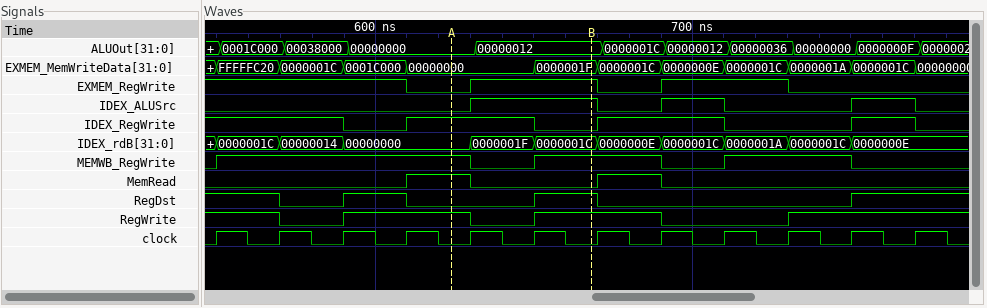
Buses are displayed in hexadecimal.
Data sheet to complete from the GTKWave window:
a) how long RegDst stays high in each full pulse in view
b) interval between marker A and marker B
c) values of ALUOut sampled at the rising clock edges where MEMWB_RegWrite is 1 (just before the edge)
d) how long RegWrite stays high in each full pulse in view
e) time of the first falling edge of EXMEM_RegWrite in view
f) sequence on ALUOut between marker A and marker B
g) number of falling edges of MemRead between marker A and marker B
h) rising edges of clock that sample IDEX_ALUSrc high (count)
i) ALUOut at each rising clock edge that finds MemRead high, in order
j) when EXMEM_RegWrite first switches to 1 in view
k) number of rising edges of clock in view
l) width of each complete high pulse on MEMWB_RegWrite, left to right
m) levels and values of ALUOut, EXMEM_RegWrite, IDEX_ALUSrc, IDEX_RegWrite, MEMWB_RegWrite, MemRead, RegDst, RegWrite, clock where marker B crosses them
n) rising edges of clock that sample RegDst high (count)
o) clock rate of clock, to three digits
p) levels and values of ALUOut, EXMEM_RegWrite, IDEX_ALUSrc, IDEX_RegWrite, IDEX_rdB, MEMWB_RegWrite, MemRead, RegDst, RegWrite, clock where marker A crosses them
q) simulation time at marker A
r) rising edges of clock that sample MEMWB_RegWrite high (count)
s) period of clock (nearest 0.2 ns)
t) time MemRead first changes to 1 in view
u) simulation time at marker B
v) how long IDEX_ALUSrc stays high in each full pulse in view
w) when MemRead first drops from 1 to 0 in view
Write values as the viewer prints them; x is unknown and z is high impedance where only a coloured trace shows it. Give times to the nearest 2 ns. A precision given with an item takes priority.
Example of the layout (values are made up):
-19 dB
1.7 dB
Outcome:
20 ns, 20 ns
44 ns
0001C000, 00038000, 00000000, 00000000, 00000012, 0000001C, 00000036, 00000000
40 ns, 40 ns
610 ns
00000000, 00000012
1
4
00000000, 0000001C
630 ns
12
80 ns, 40 ns, 40 ns
ALUOut=00000012, EXMEM_RegWrite=1, IDEX_ALUSrc=1, IDEX_RegWrite=0, MEMWB_RegWrite=1, MemRead=0, RegDst=1, RegWrite=1, clock=0
5
50.0 MHz
ALUOut=00000000, EXMEM_RegWrite=0, IDEX_ALUSrc=0, IDEX_RegWrite=1, IDEX_rdB=00000000, MEMWB_RegWrite=1, MemRead=1, RegDst=0, RegWrite=1, clock=0
624 ns
8
20 ns
610 ns
668 ns
40 ns, 20 ns, 20 ns
630 ns
